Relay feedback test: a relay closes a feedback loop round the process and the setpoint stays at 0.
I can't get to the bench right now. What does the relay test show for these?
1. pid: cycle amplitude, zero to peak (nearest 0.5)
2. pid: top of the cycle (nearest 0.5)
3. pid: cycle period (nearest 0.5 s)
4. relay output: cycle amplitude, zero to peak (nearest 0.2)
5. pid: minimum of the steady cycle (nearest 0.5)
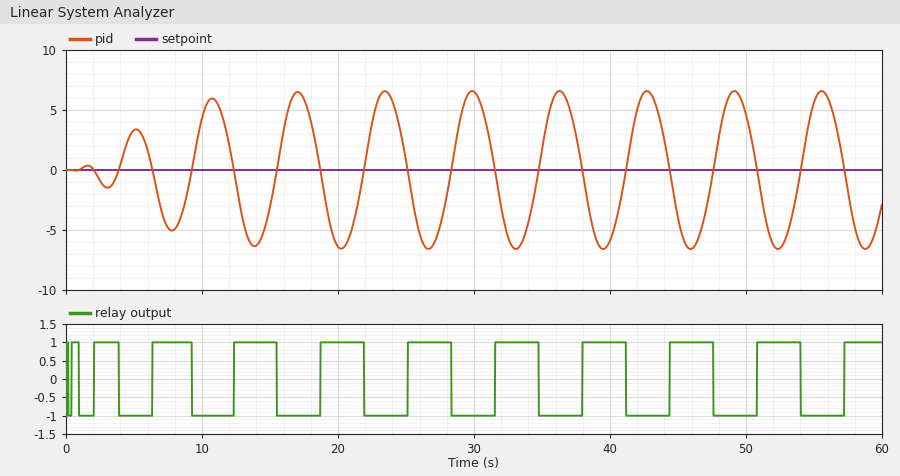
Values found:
6.5
6.5
6.5 s
1.0
-6.5
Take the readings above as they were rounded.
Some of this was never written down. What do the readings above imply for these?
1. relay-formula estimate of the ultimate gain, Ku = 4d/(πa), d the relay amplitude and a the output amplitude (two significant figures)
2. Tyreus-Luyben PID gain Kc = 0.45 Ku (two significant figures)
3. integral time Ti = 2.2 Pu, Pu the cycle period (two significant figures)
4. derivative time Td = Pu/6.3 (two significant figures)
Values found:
0.20
0.090
14 s
1.0 s
